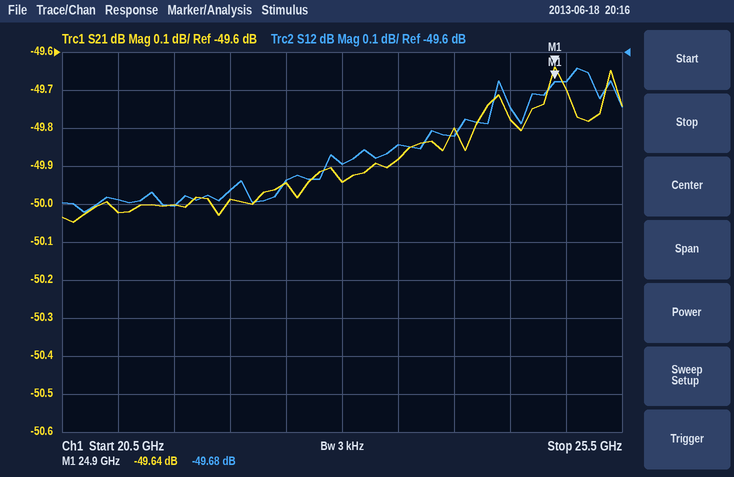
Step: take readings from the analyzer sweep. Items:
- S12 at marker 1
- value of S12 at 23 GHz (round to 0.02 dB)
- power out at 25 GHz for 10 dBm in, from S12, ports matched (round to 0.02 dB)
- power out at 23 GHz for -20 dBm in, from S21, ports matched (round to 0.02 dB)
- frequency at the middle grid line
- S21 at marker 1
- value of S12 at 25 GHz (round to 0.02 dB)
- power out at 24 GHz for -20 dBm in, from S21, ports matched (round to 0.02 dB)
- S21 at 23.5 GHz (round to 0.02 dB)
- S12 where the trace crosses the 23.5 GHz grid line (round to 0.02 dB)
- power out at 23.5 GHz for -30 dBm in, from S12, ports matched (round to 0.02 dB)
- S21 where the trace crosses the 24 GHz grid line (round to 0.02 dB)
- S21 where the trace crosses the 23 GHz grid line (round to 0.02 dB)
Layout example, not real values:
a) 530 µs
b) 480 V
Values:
a) -49.68 dB
b) -49.90 dB
c) -39.68 dBm
d) -69.94 dBm
e) 23 GHz
f) -49.64 dB
g) -49.68 dB
h) -69.80 dBm
i) -49.88 dB
j) -49.84 dB
k) -79.84 dBm
l) -49.80 dB
m) -49.94 dB
